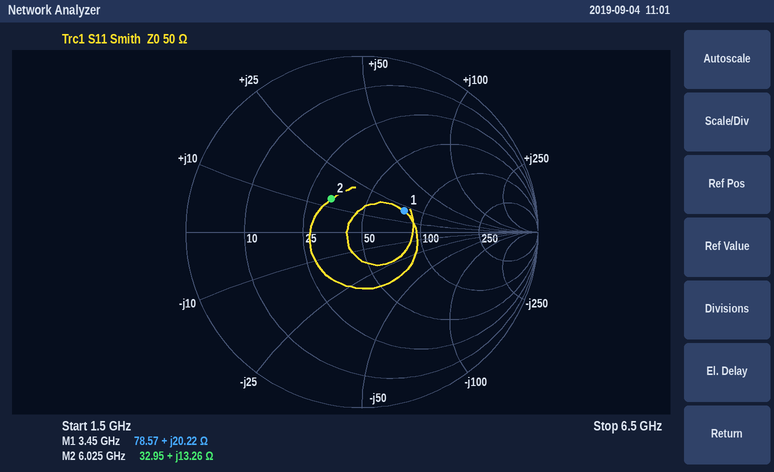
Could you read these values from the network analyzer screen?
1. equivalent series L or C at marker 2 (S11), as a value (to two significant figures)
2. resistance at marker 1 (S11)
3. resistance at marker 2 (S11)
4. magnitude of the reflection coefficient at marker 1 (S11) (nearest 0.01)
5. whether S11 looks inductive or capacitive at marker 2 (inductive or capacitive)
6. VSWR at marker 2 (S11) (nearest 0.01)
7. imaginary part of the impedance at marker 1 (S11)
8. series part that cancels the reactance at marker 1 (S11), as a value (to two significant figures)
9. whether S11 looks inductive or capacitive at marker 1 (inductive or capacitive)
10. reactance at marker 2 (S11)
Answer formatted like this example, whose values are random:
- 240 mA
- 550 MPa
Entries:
- 350 pH
- 78.57 Ω
- 32.95 Ω
- 0.27
- inductive
- 1.69
- +20.22 Ω
- 2.3 pF
- inductive
- +13.26 Ω
